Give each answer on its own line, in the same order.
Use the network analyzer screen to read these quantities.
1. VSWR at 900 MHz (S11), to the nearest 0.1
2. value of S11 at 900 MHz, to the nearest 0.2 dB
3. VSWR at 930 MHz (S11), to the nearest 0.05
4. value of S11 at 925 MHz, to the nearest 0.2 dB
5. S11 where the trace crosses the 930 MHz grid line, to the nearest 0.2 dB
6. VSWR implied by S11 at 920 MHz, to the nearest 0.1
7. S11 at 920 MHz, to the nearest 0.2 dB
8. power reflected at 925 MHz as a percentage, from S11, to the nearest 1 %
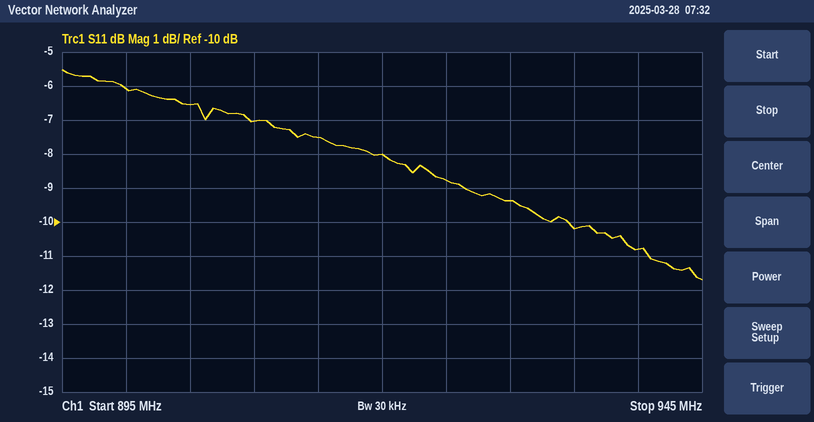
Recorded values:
3.0
-6.0 dB
2.05
-8.8 dB
-9.4 dB
2.3
-8.0 dB
13 %
